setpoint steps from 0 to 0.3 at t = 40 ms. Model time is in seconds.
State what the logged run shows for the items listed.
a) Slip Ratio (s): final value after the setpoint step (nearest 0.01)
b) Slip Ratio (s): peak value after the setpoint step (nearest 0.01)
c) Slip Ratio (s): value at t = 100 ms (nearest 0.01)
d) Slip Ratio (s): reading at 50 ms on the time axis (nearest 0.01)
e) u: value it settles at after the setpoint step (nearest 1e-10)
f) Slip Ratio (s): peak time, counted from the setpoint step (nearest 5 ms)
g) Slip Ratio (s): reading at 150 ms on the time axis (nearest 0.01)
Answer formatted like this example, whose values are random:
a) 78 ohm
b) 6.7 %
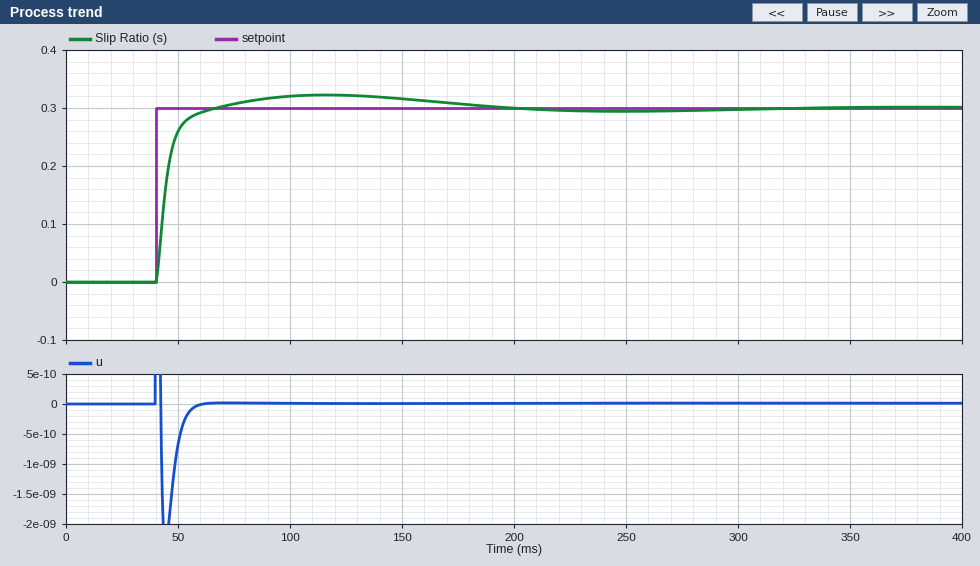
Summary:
a) 0.30
b) 0.32
c) 0.32
d) 0.26
e) 0.0000000000
f) 75 ms
g) 0.32
